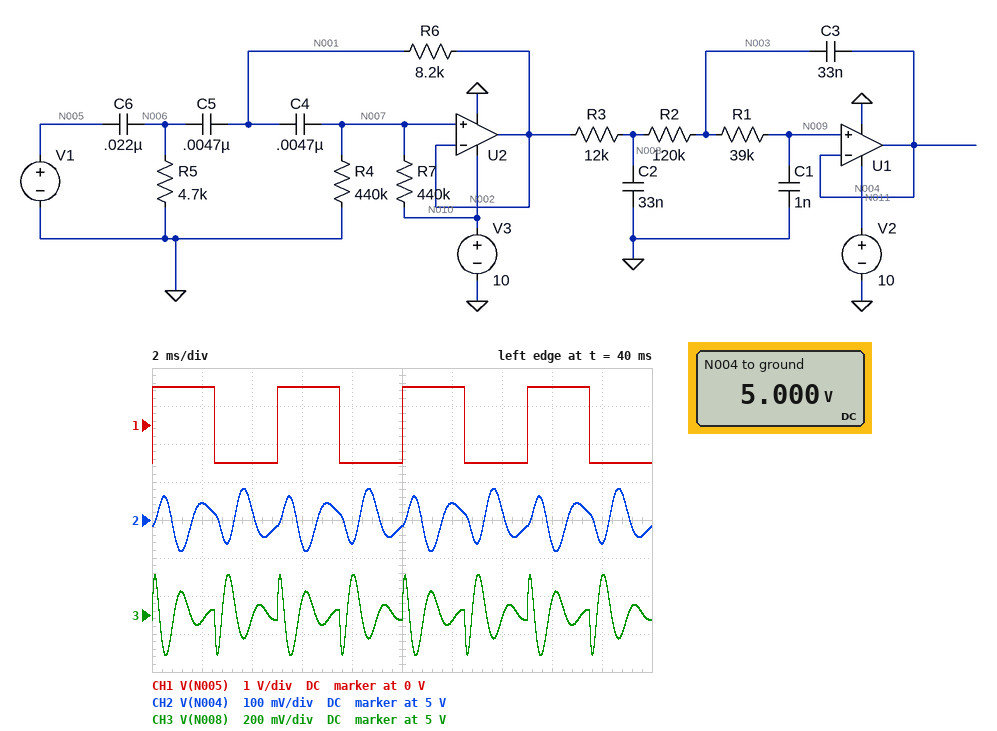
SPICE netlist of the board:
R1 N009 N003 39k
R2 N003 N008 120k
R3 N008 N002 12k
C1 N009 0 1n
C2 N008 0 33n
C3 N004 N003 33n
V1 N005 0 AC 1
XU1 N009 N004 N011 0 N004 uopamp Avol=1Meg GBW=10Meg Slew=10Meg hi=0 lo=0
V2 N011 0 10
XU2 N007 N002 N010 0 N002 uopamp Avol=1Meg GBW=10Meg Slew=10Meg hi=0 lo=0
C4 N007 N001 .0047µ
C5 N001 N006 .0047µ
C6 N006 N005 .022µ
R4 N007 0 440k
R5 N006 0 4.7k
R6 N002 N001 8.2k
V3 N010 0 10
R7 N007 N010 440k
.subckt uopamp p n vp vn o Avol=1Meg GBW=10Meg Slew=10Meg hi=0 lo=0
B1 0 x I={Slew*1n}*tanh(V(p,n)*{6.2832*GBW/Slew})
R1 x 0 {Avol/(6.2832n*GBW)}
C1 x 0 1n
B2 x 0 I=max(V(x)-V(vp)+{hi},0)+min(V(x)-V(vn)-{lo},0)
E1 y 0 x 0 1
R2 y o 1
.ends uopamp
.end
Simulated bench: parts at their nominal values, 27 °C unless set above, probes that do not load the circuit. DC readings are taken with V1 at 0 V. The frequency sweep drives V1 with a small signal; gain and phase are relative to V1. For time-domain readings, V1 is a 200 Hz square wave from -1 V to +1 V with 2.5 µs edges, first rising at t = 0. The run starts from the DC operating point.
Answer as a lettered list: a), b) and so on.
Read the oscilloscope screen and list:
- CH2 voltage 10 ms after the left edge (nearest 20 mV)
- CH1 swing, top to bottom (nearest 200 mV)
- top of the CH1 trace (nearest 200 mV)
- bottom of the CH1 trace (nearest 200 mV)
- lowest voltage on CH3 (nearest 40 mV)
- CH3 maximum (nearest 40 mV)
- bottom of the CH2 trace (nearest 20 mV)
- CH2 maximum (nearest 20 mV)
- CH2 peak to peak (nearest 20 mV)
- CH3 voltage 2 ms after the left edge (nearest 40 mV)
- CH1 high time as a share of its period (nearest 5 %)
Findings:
a) 4.98 V
b) 2.0 V
c) 1.0 V
d) -1.0 V
e) 4.80 V
f) 5.20 V
g) 4.92 V
h) 5.08 V
i) 160 mV
j) 4.96 V
k) 50 %
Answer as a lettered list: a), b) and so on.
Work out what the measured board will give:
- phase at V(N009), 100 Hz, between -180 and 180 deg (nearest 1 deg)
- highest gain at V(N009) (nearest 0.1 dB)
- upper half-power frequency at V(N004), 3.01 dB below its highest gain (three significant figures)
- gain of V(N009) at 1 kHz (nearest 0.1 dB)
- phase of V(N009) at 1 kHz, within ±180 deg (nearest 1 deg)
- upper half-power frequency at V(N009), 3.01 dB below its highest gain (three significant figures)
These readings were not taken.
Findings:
a) -118 deg
b) -16.7 dB
c) 910 Hz
d) -22.5 dB
e) -130 deg
f) 910 Hz
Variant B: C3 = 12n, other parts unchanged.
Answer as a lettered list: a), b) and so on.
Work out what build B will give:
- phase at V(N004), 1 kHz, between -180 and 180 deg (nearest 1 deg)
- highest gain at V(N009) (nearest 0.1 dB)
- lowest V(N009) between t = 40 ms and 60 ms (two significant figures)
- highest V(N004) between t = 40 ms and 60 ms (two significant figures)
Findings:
a) -101 deg
b) -6.9 dB
c) 4.8 V
d) 5.2 V
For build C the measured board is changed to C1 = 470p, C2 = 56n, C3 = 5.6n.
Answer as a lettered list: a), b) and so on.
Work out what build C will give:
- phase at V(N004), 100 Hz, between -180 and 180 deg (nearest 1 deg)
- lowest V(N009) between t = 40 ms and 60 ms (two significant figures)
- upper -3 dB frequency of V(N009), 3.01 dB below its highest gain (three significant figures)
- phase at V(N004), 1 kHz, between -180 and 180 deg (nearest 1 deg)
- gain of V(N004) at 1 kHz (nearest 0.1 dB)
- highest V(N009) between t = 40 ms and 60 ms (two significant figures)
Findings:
a) -123 deg
b) 4.8 V
c) 1.31 kHz
d) -14 deg
e) -9.2 dB
f) 5.2 V
